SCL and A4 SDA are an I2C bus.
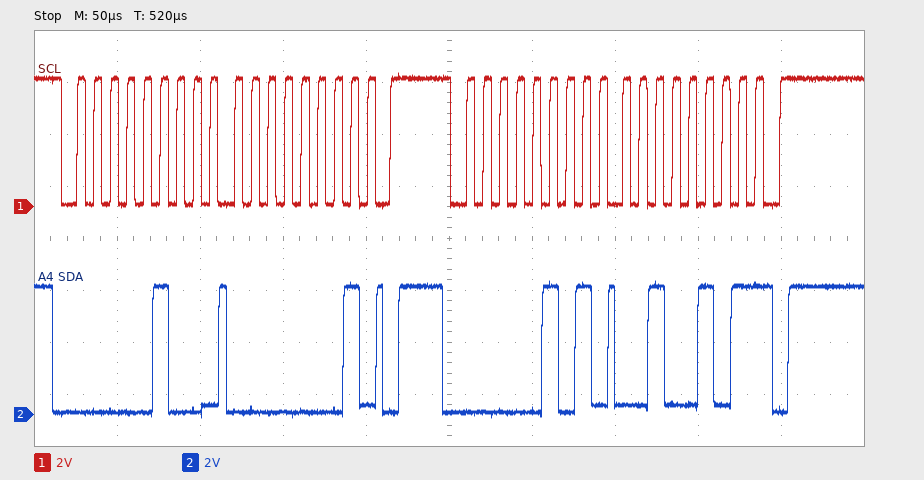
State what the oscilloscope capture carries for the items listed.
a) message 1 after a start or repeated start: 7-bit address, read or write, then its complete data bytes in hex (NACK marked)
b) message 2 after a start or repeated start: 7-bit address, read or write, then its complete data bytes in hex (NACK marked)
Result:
0x02 write: 01
0x02 read: 25 NACK
